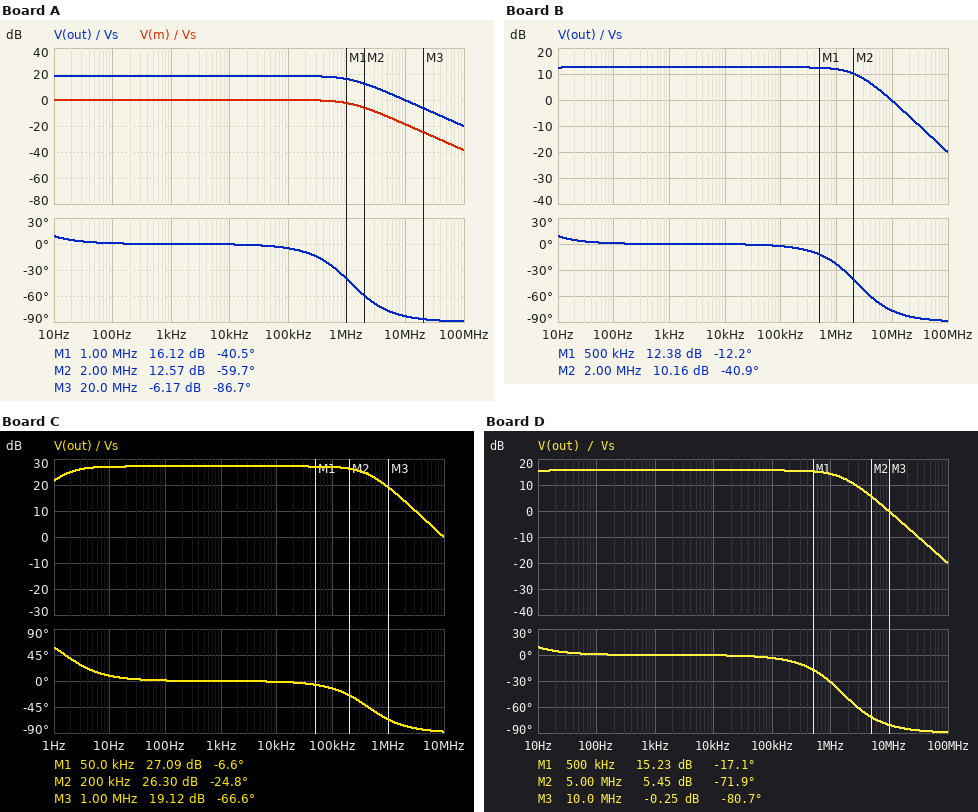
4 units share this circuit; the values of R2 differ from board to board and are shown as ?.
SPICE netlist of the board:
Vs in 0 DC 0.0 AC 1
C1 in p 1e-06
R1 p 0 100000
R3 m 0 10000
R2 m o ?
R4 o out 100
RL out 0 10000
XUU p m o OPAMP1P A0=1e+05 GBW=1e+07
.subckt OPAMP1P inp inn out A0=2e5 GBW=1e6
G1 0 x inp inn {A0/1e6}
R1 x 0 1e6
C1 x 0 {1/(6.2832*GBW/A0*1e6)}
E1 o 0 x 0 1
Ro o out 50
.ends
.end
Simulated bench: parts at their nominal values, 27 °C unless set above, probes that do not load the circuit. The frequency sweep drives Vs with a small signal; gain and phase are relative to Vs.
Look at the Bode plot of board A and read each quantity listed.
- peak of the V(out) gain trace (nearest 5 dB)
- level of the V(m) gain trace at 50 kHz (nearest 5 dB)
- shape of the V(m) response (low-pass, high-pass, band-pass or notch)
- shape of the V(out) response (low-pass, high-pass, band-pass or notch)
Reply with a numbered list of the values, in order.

1. 20 dB
2. 0 dB
3. low-pass
4. low-pass
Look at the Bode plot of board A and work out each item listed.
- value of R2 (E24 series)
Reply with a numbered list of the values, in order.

1. 75 kΩ
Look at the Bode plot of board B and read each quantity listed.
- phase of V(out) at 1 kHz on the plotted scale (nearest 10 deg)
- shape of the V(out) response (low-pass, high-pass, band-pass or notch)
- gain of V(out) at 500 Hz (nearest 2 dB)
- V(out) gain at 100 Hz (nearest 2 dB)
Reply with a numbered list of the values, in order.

1. 0 deg
2. low-pass
3. 12 dB
4. 12 dB
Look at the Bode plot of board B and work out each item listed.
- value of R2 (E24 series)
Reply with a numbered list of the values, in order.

1. 33 kΩ
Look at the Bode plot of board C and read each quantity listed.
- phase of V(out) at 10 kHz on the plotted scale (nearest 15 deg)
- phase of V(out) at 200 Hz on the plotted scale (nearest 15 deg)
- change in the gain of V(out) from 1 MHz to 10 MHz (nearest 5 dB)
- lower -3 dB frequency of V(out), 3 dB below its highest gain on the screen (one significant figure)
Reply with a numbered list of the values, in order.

1. 0 deg
2. 0 deg
3. -20 dB
4. 2 Hz
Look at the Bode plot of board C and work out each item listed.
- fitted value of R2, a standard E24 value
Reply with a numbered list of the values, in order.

1. 220 kΩ
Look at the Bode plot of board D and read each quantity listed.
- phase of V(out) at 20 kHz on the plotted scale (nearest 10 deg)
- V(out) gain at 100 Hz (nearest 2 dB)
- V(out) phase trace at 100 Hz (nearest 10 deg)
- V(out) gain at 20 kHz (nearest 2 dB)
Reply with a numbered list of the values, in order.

1. 0 deg
2. 16 dB
3. 0 deg
4. 16 dB
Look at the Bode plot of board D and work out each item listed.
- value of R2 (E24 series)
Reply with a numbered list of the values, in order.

1. 51 kΩ
